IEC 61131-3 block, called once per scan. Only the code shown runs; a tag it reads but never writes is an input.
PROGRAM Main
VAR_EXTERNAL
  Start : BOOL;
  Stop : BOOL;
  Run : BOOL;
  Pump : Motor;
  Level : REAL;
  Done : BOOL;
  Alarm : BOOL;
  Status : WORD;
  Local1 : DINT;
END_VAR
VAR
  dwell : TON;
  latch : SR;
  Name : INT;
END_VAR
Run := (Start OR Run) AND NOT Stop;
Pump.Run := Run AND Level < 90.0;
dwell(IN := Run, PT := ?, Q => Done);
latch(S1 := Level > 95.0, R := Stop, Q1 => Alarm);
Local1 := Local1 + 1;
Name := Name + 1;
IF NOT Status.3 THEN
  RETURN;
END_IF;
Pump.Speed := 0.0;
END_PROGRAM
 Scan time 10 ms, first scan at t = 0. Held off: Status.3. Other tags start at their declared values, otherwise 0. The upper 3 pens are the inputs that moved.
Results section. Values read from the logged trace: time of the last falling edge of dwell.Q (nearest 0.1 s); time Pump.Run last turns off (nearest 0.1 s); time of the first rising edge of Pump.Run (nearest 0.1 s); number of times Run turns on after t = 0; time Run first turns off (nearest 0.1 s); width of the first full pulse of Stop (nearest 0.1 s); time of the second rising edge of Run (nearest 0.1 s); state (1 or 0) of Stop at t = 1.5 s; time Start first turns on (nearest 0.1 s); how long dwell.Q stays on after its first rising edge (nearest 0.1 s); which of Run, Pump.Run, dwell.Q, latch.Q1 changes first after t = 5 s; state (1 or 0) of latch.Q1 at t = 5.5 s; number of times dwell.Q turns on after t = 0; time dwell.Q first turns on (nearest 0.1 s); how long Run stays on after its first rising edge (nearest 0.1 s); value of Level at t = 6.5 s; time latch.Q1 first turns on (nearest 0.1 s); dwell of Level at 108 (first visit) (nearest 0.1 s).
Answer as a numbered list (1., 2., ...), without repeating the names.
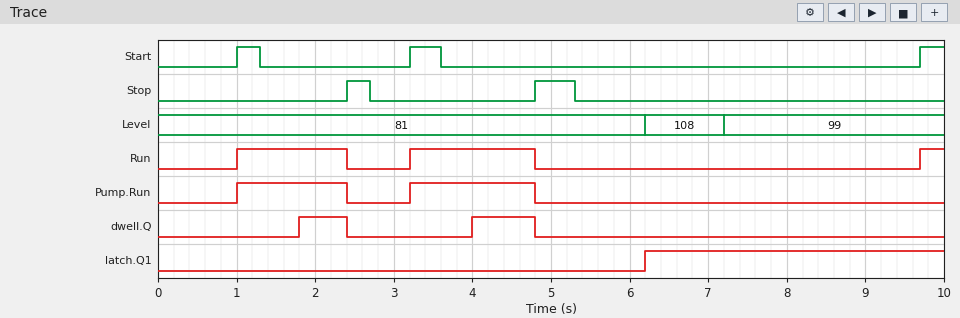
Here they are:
1. 4.8 s
2. 4.8 s
3. 1.0 s
4. 3
5. 2.4 s
6. 0.3 s
7. 3.2 s
8. 0
9. 1.0 s
10. 0.6 s
11. latch.Q1
12. 0
13. 2
14. 1.8 s
15. 1.4 s
16. 108
17. 6.2 s
18. 1.0 s
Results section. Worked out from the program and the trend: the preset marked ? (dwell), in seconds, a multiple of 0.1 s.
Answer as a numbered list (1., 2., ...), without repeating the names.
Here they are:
1. 0.8 s
